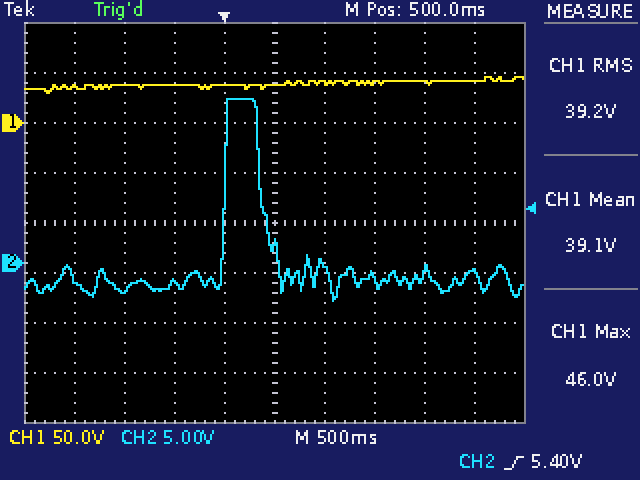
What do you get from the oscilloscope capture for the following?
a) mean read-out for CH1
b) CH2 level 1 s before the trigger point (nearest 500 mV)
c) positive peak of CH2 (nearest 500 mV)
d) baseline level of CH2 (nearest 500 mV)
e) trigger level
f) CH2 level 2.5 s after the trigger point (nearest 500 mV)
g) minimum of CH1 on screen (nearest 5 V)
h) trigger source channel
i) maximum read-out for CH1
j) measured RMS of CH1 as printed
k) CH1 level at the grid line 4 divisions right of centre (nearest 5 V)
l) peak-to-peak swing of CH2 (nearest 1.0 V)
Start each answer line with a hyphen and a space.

- 39.1 V
- -2.5 V
- 16.5 V
- -2.0 V
- 5.40 V
- -1.0 V
- 30 V
- CH2
- 46.0 V
- 39.2 V
- 40 V
- 20.0 V
